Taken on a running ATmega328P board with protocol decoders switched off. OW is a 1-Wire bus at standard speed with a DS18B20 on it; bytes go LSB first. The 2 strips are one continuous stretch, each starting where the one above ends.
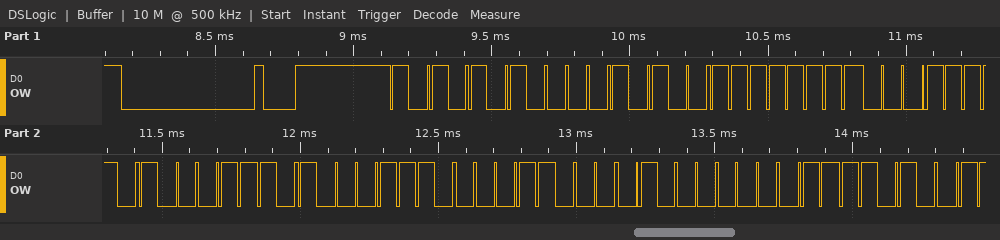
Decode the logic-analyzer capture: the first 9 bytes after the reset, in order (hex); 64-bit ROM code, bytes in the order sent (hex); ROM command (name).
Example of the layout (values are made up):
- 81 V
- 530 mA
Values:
- 55 28 FF 78 71 71 18 02 5E
- 28 FF 78 71 71 18 02 5E
- Match ROM
